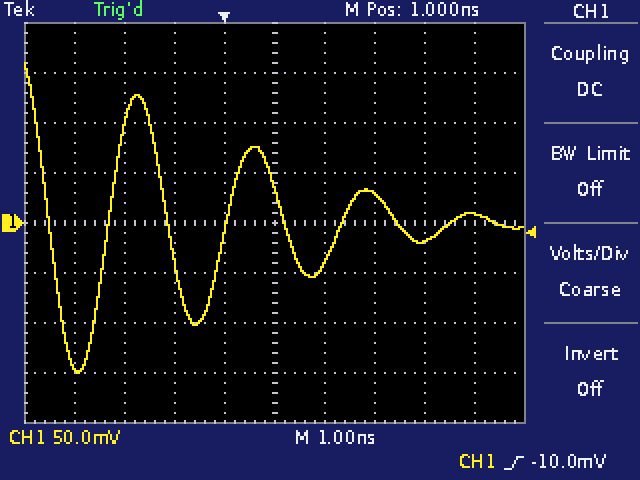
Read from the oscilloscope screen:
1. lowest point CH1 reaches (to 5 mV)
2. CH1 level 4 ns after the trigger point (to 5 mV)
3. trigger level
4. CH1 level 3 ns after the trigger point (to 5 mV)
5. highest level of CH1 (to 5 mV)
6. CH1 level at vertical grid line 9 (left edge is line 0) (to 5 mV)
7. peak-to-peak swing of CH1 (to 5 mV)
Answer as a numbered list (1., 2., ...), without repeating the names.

1. -150 mV
2. -20 mV
3. -10.0 mV
4. 30 mV
5. 160 mV
6. 10 mV
7. 310 mV
